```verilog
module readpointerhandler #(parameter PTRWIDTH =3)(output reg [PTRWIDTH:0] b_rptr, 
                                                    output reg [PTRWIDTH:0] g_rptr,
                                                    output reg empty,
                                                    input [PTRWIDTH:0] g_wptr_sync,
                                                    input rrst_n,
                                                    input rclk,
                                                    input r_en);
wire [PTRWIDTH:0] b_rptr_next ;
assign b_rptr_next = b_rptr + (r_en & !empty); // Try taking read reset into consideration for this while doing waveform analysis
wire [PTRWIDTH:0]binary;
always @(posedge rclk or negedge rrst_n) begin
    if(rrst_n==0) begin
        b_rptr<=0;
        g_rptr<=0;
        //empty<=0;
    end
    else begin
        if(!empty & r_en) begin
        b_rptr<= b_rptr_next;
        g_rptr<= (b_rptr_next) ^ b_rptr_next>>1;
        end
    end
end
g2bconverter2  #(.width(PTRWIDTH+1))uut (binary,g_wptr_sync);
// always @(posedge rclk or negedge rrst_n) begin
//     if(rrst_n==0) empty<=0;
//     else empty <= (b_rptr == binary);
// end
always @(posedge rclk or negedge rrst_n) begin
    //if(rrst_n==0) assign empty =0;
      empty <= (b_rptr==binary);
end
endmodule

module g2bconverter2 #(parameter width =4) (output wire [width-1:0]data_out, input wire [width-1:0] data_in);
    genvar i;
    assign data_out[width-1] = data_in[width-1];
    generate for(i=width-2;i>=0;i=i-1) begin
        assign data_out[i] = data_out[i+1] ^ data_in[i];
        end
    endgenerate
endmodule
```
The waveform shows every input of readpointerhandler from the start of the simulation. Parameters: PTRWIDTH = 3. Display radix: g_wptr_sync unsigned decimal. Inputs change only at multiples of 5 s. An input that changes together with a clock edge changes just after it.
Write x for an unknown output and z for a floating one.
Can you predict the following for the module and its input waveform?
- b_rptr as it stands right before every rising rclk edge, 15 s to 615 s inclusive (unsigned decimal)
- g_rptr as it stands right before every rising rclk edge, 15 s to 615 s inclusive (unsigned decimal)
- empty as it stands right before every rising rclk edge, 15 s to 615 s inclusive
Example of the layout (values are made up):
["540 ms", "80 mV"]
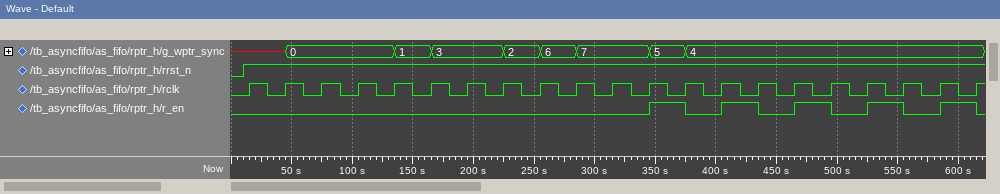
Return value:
["0, 0, 0, 0, 0, 0, 0, 0, 0, 0, 0, 0, 0, 1, 1, 2, 2, 3, 3, 4, 4", "0, 0, 0, 0, 0, 0, 0, 0, 0, 0, 0, 0, 0, 1, 1, 3, 3, 2, 2, 6, 6", "x x x 1 1 1 0 0 0 0 0 0 0 0 0 0 0 0 0 0 0"]
